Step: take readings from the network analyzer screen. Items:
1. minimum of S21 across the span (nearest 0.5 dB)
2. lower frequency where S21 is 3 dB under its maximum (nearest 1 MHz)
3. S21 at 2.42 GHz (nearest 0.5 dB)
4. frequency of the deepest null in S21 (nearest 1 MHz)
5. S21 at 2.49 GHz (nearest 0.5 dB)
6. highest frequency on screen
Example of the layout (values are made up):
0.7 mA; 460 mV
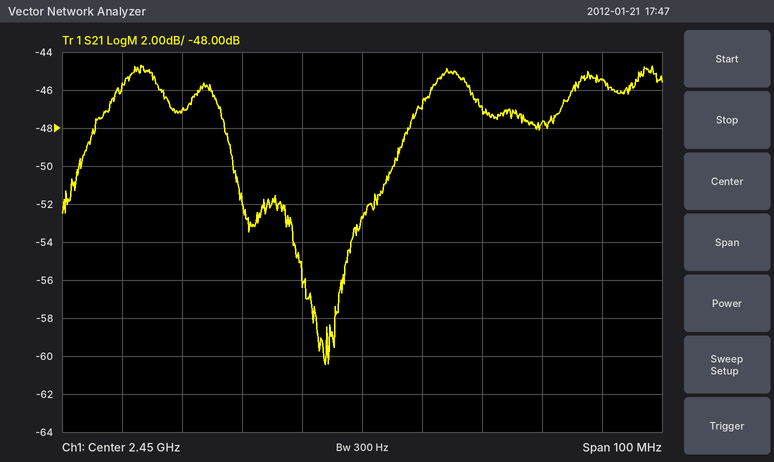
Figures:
-60.5 dB; 2.406 GHz; -47.0 dB; 2.444 GHz; -45.5 dB; 2.5 GHz
